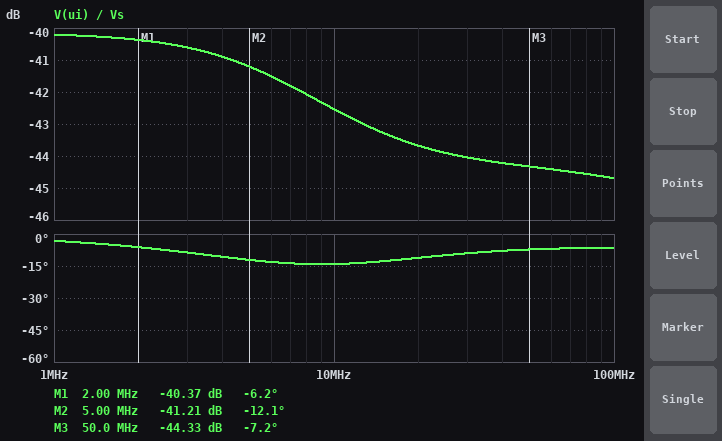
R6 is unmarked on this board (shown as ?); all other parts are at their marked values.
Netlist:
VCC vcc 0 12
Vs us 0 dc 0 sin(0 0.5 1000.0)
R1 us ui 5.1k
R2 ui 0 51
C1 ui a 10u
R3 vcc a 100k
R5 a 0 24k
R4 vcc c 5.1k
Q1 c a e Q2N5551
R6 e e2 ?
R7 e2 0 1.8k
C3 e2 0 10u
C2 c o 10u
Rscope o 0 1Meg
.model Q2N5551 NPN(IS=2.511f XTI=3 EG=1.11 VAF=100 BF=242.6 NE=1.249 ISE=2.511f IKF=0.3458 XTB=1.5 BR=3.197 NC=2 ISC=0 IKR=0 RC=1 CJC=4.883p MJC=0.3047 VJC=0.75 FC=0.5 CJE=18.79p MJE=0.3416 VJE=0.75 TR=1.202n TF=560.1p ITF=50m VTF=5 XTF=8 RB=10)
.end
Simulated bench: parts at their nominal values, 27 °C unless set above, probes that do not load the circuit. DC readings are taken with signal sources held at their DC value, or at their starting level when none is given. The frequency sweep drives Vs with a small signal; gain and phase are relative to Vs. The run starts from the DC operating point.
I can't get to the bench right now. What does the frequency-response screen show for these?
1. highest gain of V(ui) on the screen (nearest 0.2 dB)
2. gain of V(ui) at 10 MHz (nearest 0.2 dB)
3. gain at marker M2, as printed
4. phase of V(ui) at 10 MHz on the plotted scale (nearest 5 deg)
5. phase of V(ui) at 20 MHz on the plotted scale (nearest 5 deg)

-40.2 dB
-42.6 dB
-41.21 dB
-15 deg
-10 deg
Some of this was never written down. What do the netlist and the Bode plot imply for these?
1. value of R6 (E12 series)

47 Ω
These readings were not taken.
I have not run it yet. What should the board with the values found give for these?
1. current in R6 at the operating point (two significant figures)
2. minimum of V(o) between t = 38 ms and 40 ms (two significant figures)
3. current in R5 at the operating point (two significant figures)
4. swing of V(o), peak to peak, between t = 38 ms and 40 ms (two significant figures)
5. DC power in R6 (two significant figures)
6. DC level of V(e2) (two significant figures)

810 µA
-300 mV
91 µA
600 mV
31 µW
1.5 V
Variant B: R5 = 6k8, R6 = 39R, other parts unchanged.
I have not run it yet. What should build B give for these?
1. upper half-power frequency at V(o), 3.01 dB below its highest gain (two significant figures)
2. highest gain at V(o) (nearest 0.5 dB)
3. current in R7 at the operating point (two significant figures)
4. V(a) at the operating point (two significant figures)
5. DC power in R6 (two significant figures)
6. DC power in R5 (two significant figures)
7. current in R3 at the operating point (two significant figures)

12 MHz
-18.0 dB
75 µA
760 mV
220 nW
85 µW
110 µA
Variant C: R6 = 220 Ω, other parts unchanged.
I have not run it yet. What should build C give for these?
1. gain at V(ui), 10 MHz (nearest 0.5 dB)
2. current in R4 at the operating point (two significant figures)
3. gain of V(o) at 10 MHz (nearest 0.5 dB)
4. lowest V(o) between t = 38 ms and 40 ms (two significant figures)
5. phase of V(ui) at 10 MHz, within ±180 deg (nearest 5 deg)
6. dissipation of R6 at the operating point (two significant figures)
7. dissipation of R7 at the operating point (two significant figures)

-41.0 dB
740 µA
-17.5 dB
-97 mV
-5 deg
120 µW
1.0 mW
